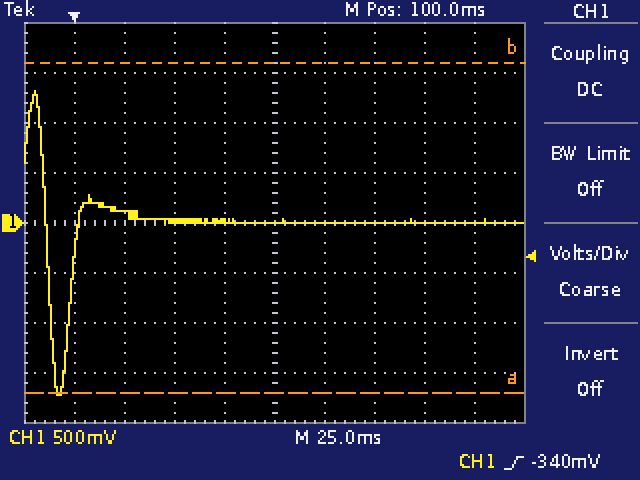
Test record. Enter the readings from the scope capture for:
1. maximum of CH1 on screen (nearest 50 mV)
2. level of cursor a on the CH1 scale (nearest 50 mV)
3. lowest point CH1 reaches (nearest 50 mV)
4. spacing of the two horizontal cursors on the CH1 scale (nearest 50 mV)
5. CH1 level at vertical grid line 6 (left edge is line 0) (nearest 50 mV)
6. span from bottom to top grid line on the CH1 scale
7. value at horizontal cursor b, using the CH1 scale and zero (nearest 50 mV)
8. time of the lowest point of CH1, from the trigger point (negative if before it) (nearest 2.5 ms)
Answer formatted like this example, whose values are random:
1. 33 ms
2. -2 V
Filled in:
1. 1.30 V
2. -1.70 V
3. -1.70 V
4. 3.30 V
5. 0 mV
6. 4 V
7. 1.60 V
8. -7.5 ms
